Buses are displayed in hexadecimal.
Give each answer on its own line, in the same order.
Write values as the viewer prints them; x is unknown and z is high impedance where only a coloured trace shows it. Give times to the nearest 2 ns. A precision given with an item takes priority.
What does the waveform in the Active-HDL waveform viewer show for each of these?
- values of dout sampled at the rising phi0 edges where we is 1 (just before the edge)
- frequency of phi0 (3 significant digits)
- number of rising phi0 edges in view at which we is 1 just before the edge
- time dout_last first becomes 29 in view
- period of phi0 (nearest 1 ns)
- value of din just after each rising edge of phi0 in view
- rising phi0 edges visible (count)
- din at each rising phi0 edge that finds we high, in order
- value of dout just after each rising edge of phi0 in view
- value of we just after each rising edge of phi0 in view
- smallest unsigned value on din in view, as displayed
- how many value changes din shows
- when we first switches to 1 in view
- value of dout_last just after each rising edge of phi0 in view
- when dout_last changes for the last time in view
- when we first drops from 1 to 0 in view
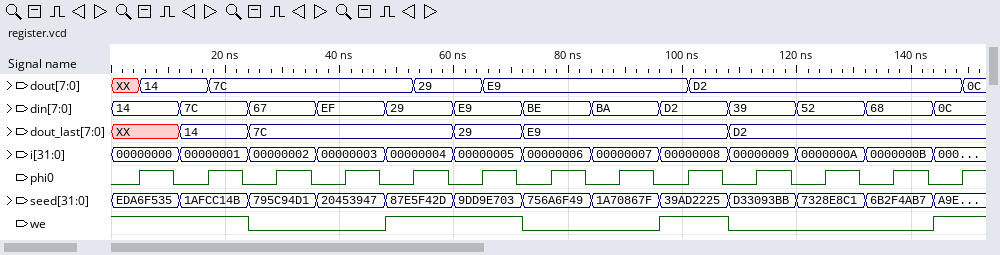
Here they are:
XX, 14, 7C, 29, E9, D2
83.3 MHz
6
60 ns
12 ns
14, 7C, 67, EF, 29, E9, BE, BA, D2, 39, 52, 68, 0C
13
14, 7C, 29, E9, D2, 0C
14, 7C, 7C, 7C, 29, E9, E9, E9, D2, D2, D2, D2, 0C
1 1 0 0 1 1 0 0 1 0 0 0 1
0C
12
48 ns
XX, 14, 7C, 7C, 7C, 29, E9, E9, E9, D2, D2, D2, D2
108 ns
24 ns
